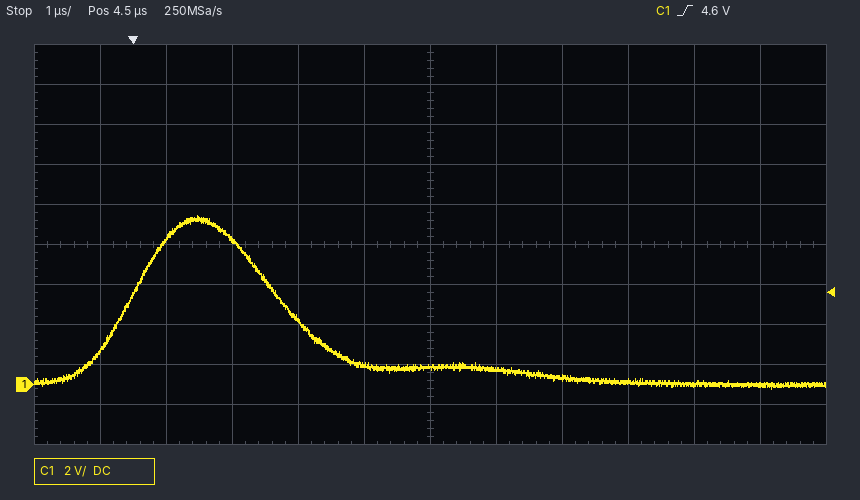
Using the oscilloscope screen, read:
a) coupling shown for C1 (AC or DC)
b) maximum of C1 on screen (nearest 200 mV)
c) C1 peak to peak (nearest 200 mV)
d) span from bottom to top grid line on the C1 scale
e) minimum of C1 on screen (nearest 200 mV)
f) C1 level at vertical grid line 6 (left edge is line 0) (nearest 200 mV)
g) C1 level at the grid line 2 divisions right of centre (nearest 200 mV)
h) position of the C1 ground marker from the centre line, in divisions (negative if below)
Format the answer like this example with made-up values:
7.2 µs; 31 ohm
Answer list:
DC; 8.4 V; 8.6 V; 20 V; -200 mV; 800 mV; 400 mV; -3.5 div
